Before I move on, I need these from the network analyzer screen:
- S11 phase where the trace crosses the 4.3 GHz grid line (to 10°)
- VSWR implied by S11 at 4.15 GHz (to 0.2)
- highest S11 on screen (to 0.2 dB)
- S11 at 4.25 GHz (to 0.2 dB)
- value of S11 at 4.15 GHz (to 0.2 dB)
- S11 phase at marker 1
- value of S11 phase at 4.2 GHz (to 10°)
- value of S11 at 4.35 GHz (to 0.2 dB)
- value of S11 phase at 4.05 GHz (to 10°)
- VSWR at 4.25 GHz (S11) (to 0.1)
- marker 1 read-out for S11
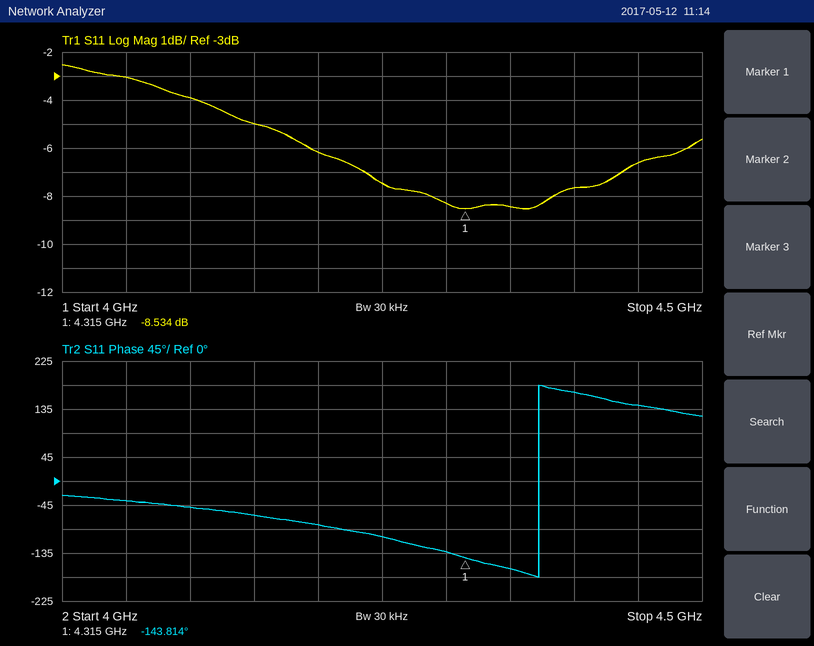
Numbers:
-130°
3.6
-2.6 dB
-7.4 dB
-5.0 dB
-143.814°
-80°
-8.4 dB
-40°
2.5
-8.534 dB
